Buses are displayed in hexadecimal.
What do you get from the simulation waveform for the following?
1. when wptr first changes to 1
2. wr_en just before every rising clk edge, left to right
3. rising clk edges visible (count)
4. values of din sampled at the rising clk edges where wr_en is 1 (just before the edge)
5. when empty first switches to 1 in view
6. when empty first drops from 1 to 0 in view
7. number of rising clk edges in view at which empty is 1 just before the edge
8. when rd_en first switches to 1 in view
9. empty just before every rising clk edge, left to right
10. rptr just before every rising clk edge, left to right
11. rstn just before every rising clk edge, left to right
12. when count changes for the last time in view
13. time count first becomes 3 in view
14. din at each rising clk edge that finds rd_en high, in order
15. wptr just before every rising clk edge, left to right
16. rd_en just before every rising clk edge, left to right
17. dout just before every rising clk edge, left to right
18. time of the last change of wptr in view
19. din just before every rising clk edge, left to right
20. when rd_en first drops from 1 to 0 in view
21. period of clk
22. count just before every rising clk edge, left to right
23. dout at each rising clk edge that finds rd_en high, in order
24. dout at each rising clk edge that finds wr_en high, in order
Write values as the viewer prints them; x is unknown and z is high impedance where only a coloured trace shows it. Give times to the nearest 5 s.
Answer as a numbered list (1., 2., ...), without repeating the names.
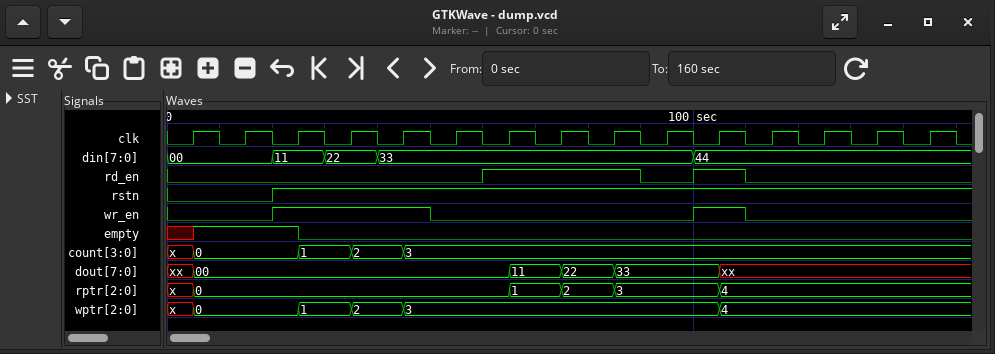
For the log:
1. 25 s
2. 0 0 1 1 1 0 0 0 0 0 1 0 0 0 0
3. 15
4. 11, 22, 33, 44
5. 5 s
6. 25 s
7. 2
8. 60 s
9. x 1 1 0 0 0 0 0 0 0 0 0 0 0 0
10. x, 0, 0, 0, 0, 0, 0, 1, 2, 3, 3, 4, 4, 4, 4
11. 0 0 1 1 1 1 1 1 1 1 1 1 1 1 1
12. 45 s
13. 45 s
14. 33, 33, 33, 44
15. x, 0, 0, 1, 2, 3, 3, 3, 3, 3, 3, 4, 4, 4, 4
16. 0 0 0 0 0 0 1 1 1 0 1 0 0 0 0
17. xx, 00, 00, 00, 00, 00, 00, 11, 22, 33, 33, xx, xx, xx, xx
18. 105 s
19. 00, 00, 11, 22, 33, 33, 33, 33, 33, 33, 44, 44, 44, 44, 44
20. 90 s
21. 10 s
22. x, 0, 0, 1, 2, 3, 3, 3, 3, 3, 3, 3, 3, 3, 3
23. 00, 11, 22, 33
24. 00, 00, 00, 33
